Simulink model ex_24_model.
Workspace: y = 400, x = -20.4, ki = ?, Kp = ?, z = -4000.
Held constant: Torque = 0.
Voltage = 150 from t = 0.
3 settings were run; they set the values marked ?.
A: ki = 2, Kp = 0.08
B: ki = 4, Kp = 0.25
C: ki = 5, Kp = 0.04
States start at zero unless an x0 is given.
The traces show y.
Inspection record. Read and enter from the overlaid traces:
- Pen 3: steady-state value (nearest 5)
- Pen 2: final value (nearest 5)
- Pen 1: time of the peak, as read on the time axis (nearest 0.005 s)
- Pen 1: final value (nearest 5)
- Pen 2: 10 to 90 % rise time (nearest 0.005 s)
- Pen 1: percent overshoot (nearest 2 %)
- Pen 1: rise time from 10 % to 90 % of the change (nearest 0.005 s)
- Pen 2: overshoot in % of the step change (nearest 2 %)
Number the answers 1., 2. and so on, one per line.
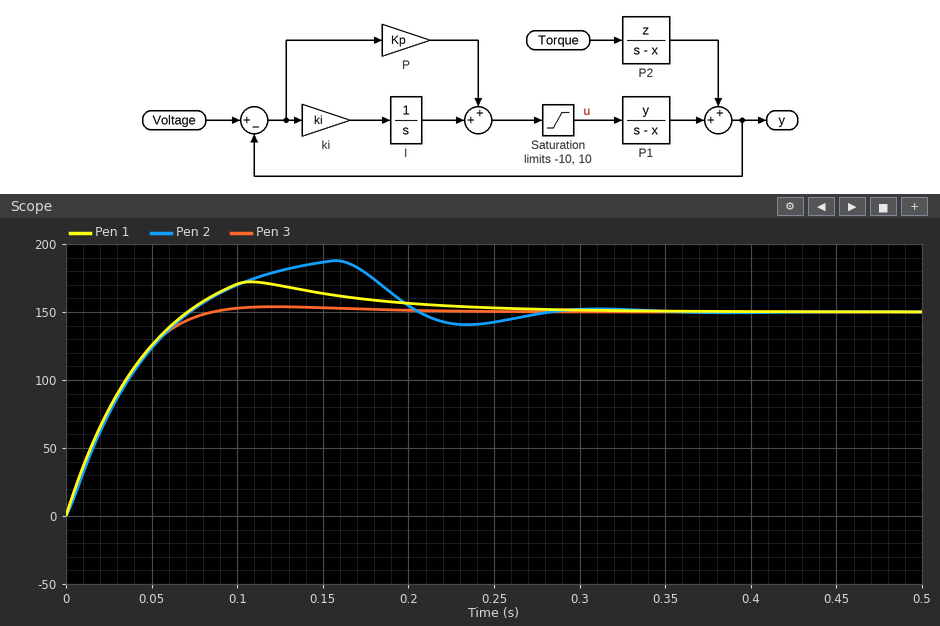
1. 150
2. 150
3. 0.110 s
4. 150
5. 0.055 s
6. 14 %
7. 0.055 s
8. 26 %
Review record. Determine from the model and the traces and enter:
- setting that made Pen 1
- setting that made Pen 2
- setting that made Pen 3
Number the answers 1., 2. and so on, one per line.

1. B
2. C
3. A
